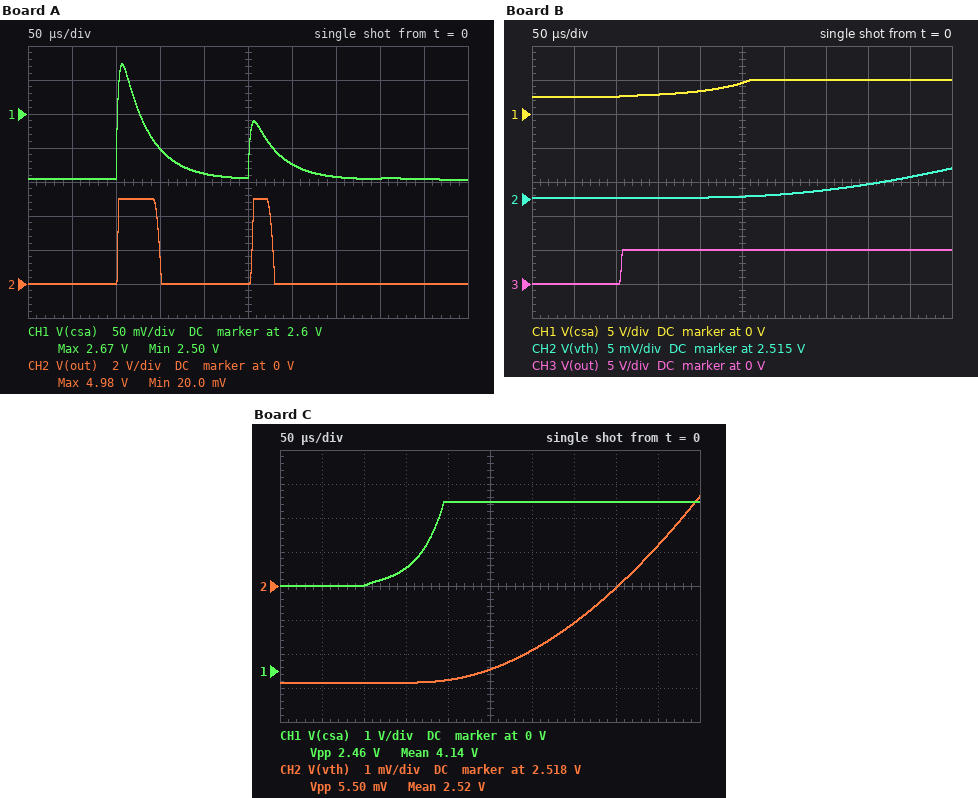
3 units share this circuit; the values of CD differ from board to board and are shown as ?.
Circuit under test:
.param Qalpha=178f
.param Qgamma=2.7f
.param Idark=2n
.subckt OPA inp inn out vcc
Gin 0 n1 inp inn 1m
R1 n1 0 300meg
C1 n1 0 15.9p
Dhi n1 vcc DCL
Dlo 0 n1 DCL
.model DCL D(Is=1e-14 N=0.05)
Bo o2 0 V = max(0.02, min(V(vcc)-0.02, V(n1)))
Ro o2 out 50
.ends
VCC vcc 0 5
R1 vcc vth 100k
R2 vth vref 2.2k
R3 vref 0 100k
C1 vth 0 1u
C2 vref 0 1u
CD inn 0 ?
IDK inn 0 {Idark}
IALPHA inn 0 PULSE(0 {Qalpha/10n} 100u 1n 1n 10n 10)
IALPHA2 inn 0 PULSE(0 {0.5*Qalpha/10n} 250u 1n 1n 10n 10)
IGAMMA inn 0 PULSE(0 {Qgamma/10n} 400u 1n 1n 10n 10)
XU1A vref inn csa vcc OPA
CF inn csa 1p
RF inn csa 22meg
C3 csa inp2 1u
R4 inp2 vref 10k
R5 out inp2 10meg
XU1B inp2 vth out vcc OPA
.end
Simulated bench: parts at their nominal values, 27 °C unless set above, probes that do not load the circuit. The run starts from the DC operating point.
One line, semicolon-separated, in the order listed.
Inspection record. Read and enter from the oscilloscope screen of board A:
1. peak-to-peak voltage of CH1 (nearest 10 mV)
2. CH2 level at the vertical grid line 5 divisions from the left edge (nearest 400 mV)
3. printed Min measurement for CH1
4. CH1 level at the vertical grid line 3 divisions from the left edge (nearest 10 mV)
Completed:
170 mV; 0 V; 2.50 V; 2.55 V
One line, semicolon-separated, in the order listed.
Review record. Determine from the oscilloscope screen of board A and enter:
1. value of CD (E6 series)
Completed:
150 pF
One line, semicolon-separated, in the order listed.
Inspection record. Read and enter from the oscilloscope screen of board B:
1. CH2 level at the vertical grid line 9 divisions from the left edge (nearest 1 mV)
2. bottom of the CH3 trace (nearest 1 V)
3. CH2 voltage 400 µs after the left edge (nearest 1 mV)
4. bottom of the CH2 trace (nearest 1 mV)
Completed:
2.518 V; 0 V; 2.517 V; 2.515 V
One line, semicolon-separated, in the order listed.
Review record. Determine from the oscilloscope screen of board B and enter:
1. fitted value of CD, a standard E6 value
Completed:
680 pF
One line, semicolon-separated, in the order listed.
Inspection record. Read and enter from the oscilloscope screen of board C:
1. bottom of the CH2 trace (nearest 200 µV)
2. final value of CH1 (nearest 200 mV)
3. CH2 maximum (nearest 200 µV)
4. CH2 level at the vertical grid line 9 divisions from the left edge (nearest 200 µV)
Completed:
2.5152 V; 5.0 V; 2.5206 V; 2.5192 V
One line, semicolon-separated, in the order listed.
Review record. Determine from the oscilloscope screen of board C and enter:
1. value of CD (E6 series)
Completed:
1 nF
